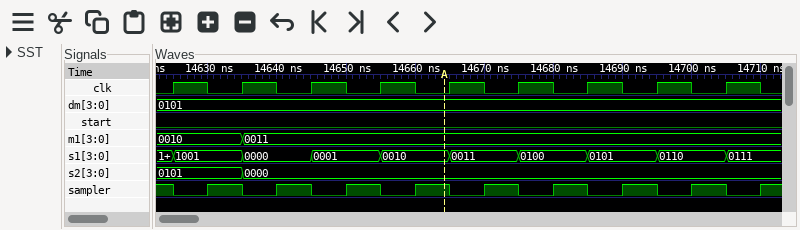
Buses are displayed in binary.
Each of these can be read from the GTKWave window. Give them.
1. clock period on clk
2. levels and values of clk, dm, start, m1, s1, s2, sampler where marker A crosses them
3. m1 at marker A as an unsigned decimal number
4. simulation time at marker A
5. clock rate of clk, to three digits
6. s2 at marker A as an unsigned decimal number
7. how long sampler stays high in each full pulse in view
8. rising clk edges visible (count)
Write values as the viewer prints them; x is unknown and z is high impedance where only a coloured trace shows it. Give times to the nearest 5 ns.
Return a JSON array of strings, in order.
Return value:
["10 ns", "clk=0, dm=0101, start=0, m1=0011, s1=0010, s2=0000, sampler=1", "3", "14665 ns", "100 MHz", "0", "5 ns, 5 ns, 5 ns, 5 ns, 5 ns, 5 ns, 5 ns, 5 ns", "9"]
